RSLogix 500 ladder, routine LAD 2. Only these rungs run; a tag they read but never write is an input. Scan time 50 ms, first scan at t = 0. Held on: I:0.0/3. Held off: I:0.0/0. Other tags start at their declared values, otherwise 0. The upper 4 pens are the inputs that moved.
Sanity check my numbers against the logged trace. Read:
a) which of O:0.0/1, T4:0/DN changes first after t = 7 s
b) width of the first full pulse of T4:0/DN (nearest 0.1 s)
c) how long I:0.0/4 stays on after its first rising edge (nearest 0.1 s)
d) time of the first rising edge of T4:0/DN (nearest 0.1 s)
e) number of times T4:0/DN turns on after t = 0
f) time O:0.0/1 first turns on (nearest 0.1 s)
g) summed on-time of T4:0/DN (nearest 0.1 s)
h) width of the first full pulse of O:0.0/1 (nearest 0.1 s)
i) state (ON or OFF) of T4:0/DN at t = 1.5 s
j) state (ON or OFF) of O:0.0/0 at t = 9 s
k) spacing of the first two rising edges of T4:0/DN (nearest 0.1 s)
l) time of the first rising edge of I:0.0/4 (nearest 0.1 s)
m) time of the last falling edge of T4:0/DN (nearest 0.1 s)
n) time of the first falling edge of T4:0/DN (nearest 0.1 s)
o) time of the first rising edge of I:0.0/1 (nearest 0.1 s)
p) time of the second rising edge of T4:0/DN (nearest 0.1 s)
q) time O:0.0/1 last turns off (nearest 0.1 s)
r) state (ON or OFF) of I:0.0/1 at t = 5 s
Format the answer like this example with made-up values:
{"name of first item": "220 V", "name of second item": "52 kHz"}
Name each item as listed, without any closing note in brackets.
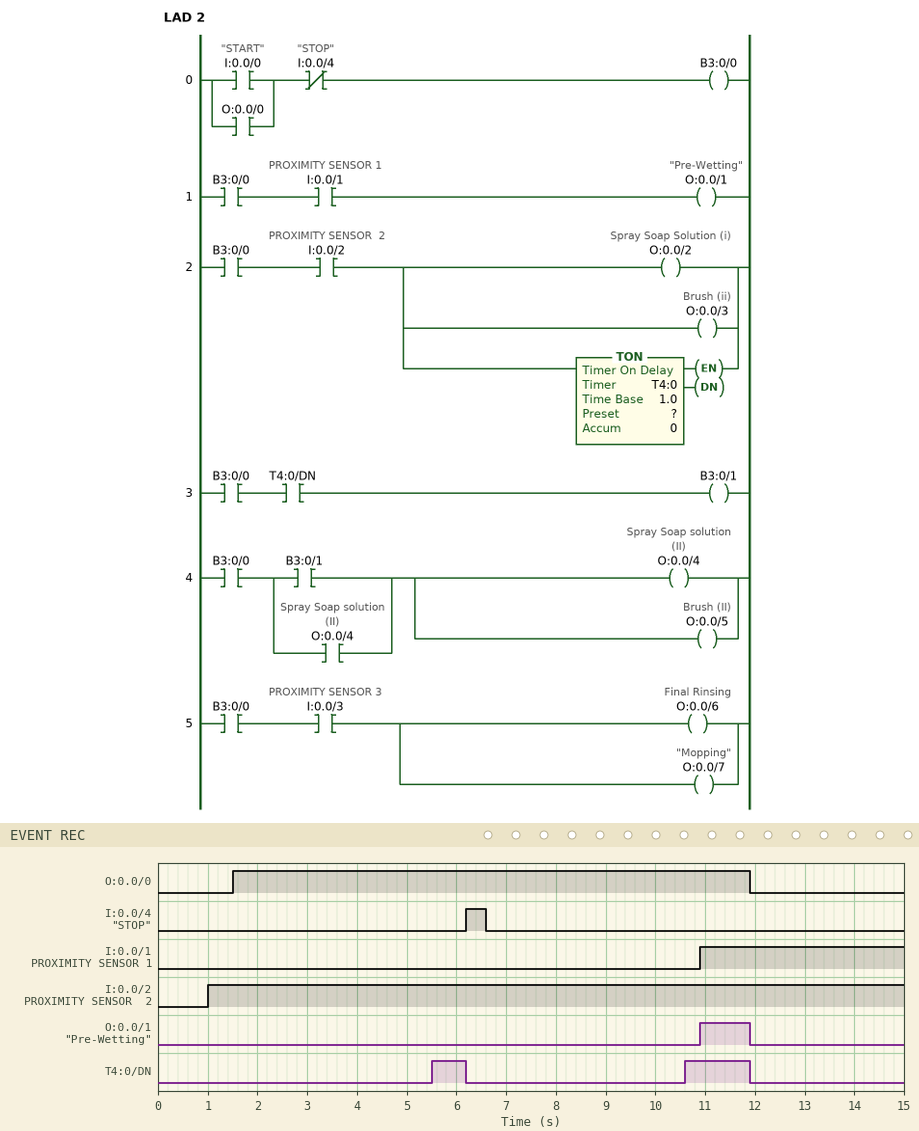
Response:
{"which of O:0.0/1, T4:0/DN changes first after t = 7 s": "T4:0/DN", "width of the first full pulse of T4:0/DN": "0.7 s", "how long I:0.0/4 stays on after its first rising edge": "0.4 s", "time of the first rising edge of T4:0/DN": "5.5 s", "number of times T4:0/DN turns on after t = 0": "2", "time O:0.0/1 first turns on": "10.9 s", "summed on-time of T4:0/DN": "2.0 s", "width of the first full pulse of O:0.0/1": "1.0 s", "state (ON or OFF) of T4:0/DN at t = 1.5 s": "OFF", "state (ON or OFF) of O:0.0/0 at t = 9 s": "ON", "spacing of the first two rising edges of T4:0/DN": "5.1 s", "time of the first rising edge of I:0.0/4": "6.2 s", "time of the last falling edge of T4:0/DN": "11.9 s", "time of the first falling edge of T4:0/DN": "6.2 s", "time of the first rising edge of I:0.0/1": "10.9 s", "time of the second rising edge of T4:0/DN": "10.6 s", "time O:0.0/1 last turns off": "11.9 s", "state (ON or OFF) of I:0.0/1 at t = 5 s": "OFF"}
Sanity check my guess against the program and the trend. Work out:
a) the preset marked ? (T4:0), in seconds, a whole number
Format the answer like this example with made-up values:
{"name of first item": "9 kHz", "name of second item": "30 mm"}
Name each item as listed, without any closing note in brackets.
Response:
{"the preset marked ? (T4:0), in seconds, a whole number": "4 s"}
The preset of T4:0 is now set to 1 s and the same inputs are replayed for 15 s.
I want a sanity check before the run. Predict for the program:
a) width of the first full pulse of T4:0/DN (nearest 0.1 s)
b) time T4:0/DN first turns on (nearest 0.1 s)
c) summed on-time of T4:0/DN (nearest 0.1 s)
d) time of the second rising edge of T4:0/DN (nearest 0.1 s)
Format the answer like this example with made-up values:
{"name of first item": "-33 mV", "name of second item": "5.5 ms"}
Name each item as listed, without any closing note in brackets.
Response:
{"width of the first full pulse of T4:0/DN": "3.7 s", "time T4:0/DN first turns on": "2.5 s", "summed on-time of T4:0/DN": "8.0 s", "time of the second rising edge of T4:0/DN": "7.6 s"}
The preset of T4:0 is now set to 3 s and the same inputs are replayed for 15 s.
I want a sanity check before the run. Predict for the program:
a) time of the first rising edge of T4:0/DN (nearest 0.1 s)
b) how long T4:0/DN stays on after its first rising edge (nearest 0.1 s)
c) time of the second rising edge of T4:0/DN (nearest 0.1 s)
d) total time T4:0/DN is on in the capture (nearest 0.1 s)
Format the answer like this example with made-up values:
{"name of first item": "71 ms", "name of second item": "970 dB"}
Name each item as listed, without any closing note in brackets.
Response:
{"time of the first rising edge of T4:0/DN": "4.5 s", "how long T4:0/DN stays on after its first rising edge": "1.7 s", "time of the second rising edge of T4:0/DN": "9.6 s", "total time T4:0/DN is on in the capture": "4.0 s"}
